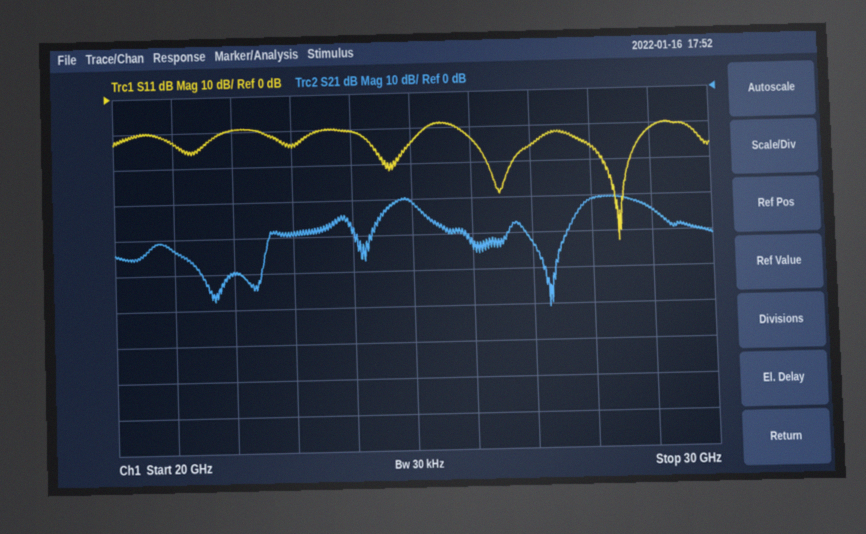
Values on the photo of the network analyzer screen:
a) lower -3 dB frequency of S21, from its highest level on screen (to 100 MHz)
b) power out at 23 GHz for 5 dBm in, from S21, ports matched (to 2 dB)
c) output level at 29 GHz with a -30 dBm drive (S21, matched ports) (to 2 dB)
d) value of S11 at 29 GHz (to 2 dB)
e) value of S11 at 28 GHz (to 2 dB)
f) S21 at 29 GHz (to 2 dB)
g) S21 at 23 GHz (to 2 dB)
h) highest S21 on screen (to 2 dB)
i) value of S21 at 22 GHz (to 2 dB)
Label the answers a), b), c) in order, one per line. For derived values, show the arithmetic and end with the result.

a) 24.6 GHz
b) 5 dBm + (-40 dB) = -34 dBm
c) -30 dBm + (-34 dB) = -64 dBm
d) -12 dB
e) -16 dB
f) -34 dB
g) -40 dB
h) -30 dB
i) -50 dB
